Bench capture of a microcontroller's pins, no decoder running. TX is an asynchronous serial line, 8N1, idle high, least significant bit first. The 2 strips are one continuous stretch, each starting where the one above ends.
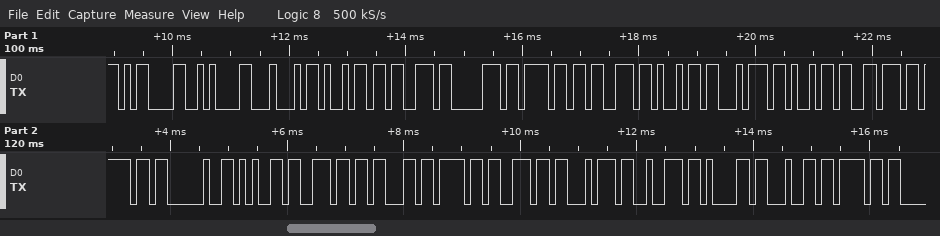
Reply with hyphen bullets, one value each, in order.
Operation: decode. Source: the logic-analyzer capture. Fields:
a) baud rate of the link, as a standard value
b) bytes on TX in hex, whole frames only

- 9600 baud
- 0D 0A 44 69 73 70 6F 73 69 74 69 76 6F 20 65 6E 63 6F 6E 74 72 61 64 6F
